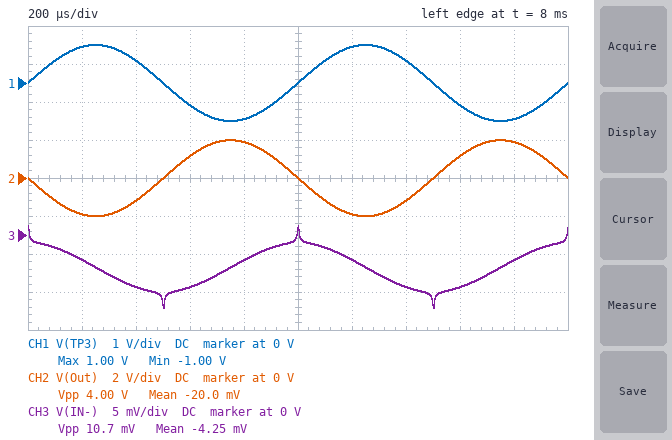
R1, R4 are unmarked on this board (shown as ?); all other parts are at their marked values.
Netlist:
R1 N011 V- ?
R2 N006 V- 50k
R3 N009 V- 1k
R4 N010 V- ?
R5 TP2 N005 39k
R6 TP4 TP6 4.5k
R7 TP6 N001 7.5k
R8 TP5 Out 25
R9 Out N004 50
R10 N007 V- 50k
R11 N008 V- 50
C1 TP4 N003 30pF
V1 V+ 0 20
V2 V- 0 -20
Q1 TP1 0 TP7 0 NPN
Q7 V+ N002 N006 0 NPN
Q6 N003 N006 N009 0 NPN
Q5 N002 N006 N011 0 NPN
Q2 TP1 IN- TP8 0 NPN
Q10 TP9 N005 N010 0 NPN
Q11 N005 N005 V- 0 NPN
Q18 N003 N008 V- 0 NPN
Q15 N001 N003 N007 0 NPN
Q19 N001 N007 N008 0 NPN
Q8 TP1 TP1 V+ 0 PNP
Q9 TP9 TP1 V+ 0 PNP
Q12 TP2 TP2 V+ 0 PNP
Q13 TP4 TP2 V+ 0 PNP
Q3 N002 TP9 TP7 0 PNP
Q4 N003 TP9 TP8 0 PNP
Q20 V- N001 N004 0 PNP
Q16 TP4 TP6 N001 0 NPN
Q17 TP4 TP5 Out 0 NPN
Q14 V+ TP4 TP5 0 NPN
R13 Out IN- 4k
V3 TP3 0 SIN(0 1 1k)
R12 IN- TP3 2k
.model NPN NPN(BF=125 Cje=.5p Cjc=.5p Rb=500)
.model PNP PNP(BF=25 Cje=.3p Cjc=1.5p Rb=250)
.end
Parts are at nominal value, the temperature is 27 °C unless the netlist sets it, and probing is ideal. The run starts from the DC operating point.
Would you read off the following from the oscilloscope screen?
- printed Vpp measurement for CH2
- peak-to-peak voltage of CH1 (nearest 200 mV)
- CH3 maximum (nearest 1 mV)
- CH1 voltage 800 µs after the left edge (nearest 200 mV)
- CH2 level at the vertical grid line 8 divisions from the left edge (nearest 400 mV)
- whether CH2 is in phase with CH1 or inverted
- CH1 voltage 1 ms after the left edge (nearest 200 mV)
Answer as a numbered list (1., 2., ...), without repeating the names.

1. 4.00 V
2. 2.0 V
3. 1 mV
4. -1.0 V
5. 1.2 V
6. inverted
7. 0 V
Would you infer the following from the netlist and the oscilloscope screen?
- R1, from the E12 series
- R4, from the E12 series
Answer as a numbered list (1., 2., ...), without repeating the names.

1. 560 Ω
2. 8.2 kΩ
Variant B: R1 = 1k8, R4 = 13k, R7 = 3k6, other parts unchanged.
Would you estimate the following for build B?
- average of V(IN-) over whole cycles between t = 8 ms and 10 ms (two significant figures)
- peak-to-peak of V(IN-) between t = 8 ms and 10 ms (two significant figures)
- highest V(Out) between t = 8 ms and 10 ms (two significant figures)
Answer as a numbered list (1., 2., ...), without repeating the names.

1. 6.7 mV
2. 7.5 mV
3. 2.0 V
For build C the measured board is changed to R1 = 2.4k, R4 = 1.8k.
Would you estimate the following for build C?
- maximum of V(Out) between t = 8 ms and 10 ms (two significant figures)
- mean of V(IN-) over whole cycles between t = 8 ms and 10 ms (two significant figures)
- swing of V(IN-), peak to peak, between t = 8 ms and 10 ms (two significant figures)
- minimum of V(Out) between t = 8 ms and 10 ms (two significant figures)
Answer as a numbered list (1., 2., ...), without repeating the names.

1. 2.1 V
2. 26 mV
3. 2.2 mV
4. -1.9 V
